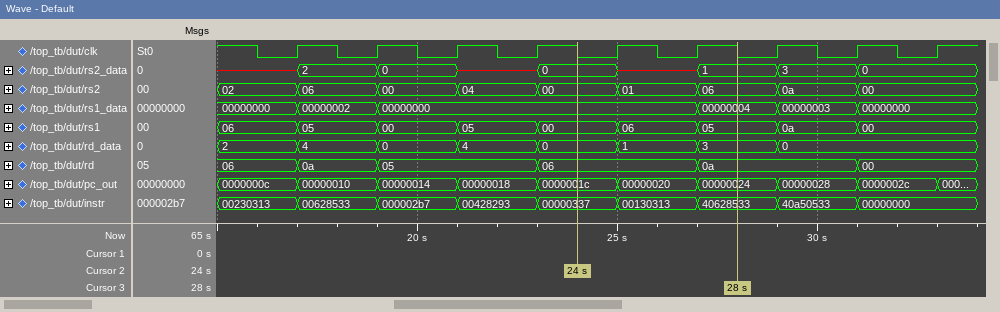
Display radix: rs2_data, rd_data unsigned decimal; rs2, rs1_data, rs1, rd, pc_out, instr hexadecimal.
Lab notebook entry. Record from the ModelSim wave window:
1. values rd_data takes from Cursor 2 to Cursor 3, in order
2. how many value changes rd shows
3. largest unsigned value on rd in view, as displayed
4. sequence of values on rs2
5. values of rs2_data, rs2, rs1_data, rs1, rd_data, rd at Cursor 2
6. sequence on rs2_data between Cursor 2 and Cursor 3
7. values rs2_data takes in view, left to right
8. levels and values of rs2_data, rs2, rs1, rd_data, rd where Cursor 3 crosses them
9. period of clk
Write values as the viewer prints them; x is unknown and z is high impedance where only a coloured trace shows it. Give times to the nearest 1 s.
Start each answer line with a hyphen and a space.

- 0, 1, 3
- 5
- 0a
- 02, 06, 00, 04, 00, 01, 06, 0a, 00
- rs2_data=0, rs2=00, rs1_data=00000000, rs1=00, rd_data=0, rd=06
- 0, x, 1
- x, 2, 0, x, 0, x, 1, 3, 0
- rs2_data=1, rs2=06, rs1=05, rd_data=3, rd=0a
- 2 s
